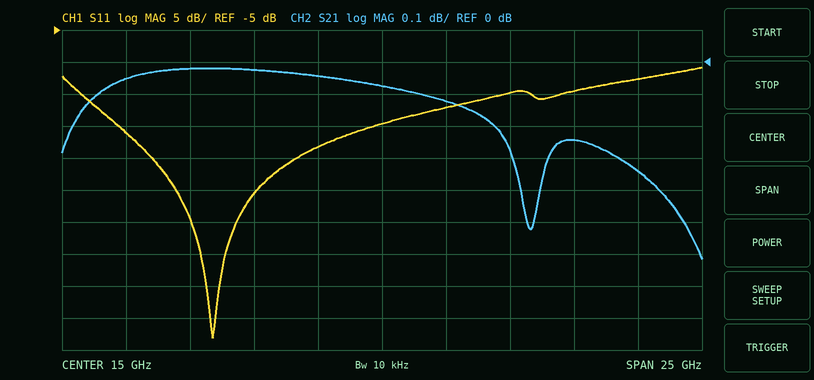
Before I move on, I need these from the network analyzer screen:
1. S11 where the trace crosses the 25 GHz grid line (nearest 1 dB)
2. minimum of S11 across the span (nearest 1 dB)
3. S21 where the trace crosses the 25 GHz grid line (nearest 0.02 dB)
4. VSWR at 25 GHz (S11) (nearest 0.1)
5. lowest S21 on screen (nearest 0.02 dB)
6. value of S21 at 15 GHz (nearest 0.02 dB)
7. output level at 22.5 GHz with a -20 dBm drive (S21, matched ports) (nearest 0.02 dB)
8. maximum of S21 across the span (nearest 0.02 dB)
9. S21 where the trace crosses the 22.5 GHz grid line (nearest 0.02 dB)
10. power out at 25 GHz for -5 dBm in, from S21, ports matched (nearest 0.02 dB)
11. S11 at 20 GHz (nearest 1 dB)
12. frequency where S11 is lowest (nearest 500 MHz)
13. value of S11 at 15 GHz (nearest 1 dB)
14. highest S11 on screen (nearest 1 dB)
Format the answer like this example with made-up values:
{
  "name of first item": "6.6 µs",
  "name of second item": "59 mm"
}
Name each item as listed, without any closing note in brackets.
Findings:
{
  "S11 where the trace crosses the 25 GHz grid line": "-13 dB",
  "minimum of S11 across the span": "-53 dB",
  "S21 where the trace crosses the 25 GHz grid line": "-0.34 dB",
  "VSWR at 25 GHz (S11)": "1.6",
  "lowest S21 on screen": "-0.62 dB",
  "value of S21 at 15 GHz": "-0.08 dB",
  "output level at 22.5 GHz with a -20 dBm drive (S21, matched ports)": "-20.24 dBm",
  "maximum of S21 across the span": "-0.02 dB",
  "S21 where the trace crosses the 22.5 GHz grid line": "-0.24 dB",
  "power out at 25 GHz for -5 dBm in, from S21, ports matched": "-5.34 dBm",
  "S11 at 20 GHz": "-15 dB",
  "frequency where S11 is lowest": "8.5 GHz",
  "value of S11 at 15 GHz": "-20 dB",
  "highest S11 on screen": "-11 dB"
}
